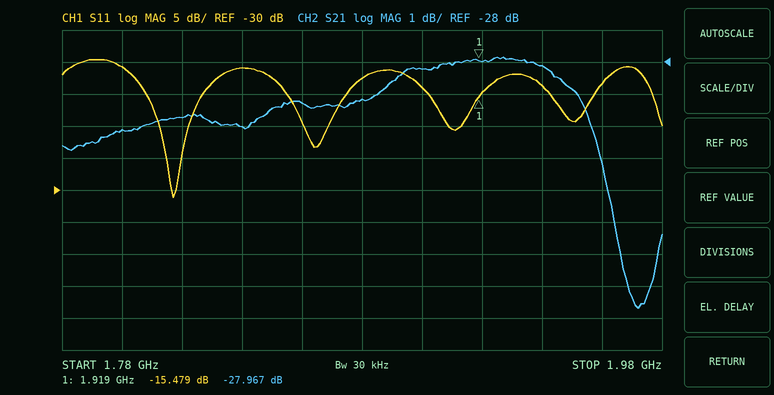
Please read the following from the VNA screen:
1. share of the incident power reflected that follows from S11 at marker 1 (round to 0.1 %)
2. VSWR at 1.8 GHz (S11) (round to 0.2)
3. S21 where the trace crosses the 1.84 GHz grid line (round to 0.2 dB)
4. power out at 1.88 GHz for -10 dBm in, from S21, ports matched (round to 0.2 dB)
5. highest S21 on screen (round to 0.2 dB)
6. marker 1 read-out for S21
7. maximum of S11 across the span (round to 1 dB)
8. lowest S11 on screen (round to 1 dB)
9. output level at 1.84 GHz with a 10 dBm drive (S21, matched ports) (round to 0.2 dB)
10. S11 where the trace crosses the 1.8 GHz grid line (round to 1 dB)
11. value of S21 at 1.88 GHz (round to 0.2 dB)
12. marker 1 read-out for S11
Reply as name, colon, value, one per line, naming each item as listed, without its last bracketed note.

share of the incident power reflected that follows from S11 at marker 1: 2.8 %
VSWR at 1.8 GHz (S11): 1.8
S21 where the trace crosses the 1.84 GHz grid line: -30.0 dB
power out at 1.88 GHz for -10 dBm in, from S21, ports matched: -39.2 dBm
highest S21 on screen: -27.8 dB
marker 1 read-out for S21: -27.967 dB
maximum of S11 across the span: -10 dB
lowest S11 on screen: -31 dB
output level at 1.84 GHz with a 10 dBm drive (S21, matched ports): -20.0 dBm
S11 where the trace crosses the 1.8 GHz grid line: -11 dB
value of S21 at 1.88 GHz: -29.2 dB
marker 1 read-out for S11: -15.479 dB
